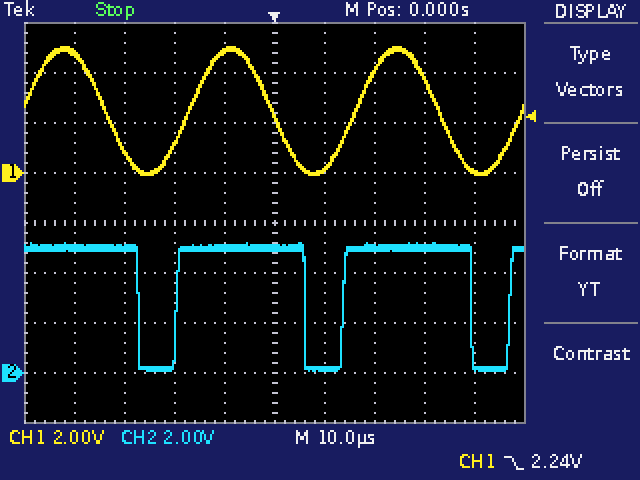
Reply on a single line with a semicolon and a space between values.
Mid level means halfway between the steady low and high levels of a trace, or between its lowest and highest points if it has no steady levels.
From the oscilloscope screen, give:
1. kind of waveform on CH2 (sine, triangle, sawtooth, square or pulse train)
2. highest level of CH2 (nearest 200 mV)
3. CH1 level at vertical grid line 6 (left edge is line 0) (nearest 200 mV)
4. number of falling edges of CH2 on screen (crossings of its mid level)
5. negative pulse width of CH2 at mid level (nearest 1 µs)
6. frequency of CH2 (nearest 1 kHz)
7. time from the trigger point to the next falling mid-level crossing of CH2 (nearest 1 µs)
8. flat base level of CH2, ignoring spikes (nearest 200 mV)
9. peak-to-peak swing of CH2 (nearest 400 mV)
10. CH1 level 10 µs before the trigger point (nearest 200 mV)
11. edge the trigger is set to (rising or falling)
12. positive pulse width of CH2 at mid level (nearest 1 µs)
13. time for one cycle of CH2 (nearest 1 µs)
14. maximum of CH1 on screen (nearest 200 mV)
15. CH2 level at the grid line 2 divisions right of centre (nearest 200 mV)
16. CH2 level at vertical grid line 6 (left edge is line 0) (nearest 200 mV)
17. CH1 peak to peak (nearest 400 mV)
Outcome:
pulse train; 5.2 V; 200 mV; 3; 8 µs; 30 kHz; 6 µs; 200 mV; 5.2 V; 4.8 V; falling; 26 µs; 33 µs; 5.0 V; 5.0 V; 200 mV; 5.2 V
